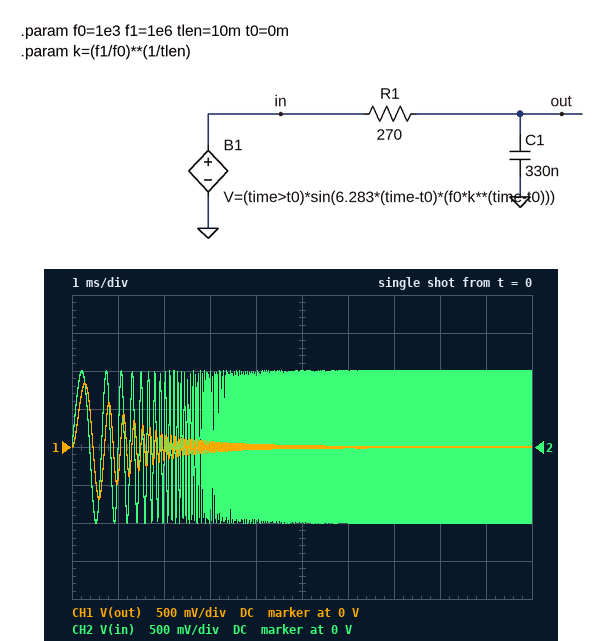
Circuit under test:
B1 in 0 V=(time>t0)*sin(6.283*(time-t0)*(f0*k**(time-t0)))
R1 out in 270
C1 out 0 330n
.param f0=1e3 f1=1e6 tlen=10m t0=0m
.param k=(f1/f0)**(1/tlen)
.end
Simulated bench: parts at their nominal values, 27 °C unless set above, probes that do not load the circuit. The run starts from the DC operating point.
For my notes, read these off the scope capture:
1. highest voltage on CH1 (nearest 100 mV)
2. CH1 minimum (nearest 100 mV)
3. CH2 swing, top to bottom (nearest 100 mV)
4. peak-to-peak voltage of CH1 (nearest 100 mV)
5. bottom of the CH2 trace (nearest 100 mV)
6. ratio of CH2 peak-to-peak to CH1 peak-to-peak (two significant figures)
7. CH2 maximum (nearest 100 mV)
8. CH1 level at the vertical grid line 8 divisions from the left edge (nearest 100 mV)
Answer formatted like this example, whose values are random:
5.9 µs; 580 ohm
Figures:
800 mV; -700 mV; 2.0 V; 1.5 V; -1.0 V; 1.3; 1.0 V; 0 V
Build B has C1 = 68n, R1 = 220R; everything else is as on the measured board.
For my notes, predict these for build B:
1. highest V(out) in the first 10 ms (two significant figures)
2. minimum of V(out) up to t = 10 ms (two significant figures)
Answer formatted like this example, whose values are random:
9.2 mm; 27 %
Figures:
990 mV; -980 mV
